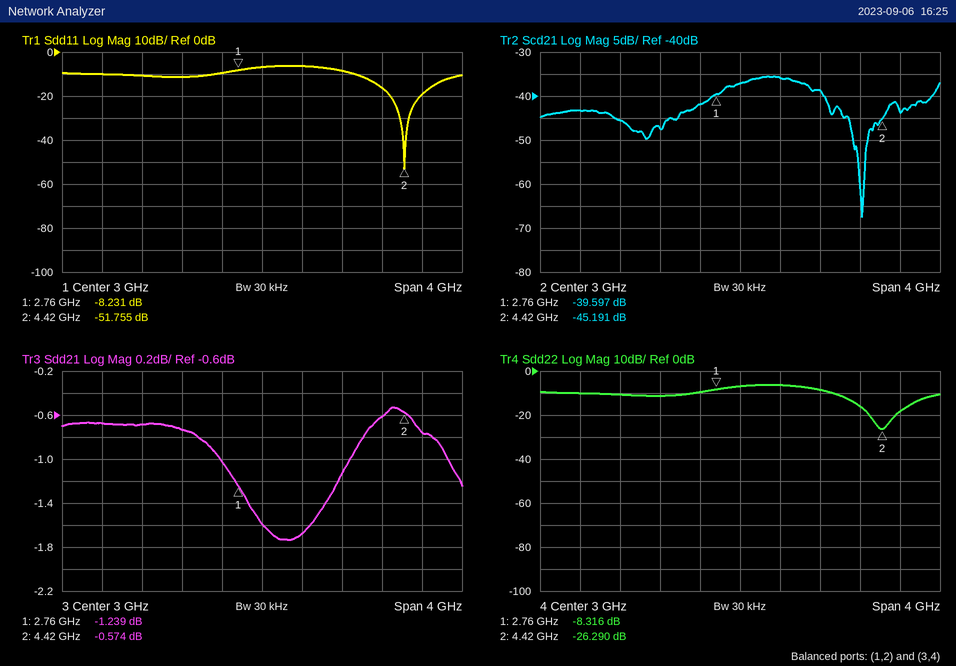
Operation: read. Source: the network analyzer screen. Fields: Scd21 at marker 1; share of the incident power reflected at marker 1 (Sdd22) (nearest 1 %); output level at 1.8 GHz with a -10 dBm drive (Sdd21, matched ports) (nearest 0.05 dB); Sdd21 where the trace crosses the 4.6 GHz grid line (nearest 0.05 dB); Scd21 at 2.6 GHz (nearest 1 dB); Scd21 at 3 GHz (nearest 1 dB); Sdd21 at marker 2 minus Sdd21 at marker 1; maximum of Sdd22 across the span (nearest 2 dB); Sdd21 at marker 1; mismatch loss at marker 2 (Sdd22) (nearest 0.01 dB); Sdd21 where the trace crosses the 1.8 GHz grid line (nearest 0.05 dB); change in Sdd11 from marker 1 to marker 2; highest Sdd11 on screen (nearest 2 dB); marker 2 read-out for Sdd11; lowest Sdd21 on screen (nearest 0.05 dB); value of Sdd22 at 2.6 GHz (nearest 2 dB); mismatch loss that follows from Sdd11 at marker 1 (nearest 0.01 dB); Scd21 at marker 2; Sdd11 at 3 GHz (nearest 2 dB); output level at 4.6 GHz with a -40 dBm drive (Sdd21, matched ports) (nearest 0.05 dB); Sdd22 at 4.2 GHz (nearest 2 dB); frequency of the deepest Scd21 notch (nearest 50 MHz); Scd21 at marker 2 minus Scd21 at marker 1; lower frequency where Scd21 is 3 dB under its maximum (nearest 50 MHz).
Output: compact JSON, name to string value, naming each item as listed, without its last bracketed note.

{"Scd21 at marker 1": "-39.597 dB", "share of the incident power reflected at marker 1 (Sdd22)": "15 %", "output level at 1.8 GHz with a -10 dBm drive (Sdd21, matched ports)": "-10.70 dBm", "Sdd21 where the trace crosses the 4.6 GHz grid line": "-0.75 dB", "Scd21 at 2.6 GHz": "-42 dB", "Scd21 at 3 GHz": "-37 dB", "Sdd21 at marker 2 minus Sdd21 at marker 1": "0.665 dB", "maximum of Sdd22 across the span": "-6 dB", "Sdd21 at marker 1": "-1.239 dB", "mismatch loss at marker 2 (Sdd22)": "0.01 dB", "Sdd21 where the trace crosses the 1.8 GHz grid line": "-0.70 dB", "change in Sdd11 from marker 1 to marker 2": "-43.524 dB", "highest Sdd11 on screen": "-6 dB", "marker 2 read-out for Sdd11": "-51.755 dB", "lowest Sdd21 on screen": "-1.75 dB", "value of Sdd22 at 2.6 GHz": "-10 dB", "mismatch loss that follows from Sdd11 at marker 1": "0.71 dB", "Scd21 at marker 2": "-45.191 dB", "Sdd11 at 3 GHz": "-6 dB", "output level at 4.6 GHz with a -40 dBm drive (Sdd21, matched ports)": "-40.75 dBm", "Sdd22 at 4.2 GHz": "-16 dB", "frequency of the deepest Scd21 notch": "4.20 GHz", "Scd21 at marker 2 minus Scd21 at marker 1": "-5.594 dB", "lower frequency where Scd21 is 3 dB under its maximum": "2.85 GHz"}
